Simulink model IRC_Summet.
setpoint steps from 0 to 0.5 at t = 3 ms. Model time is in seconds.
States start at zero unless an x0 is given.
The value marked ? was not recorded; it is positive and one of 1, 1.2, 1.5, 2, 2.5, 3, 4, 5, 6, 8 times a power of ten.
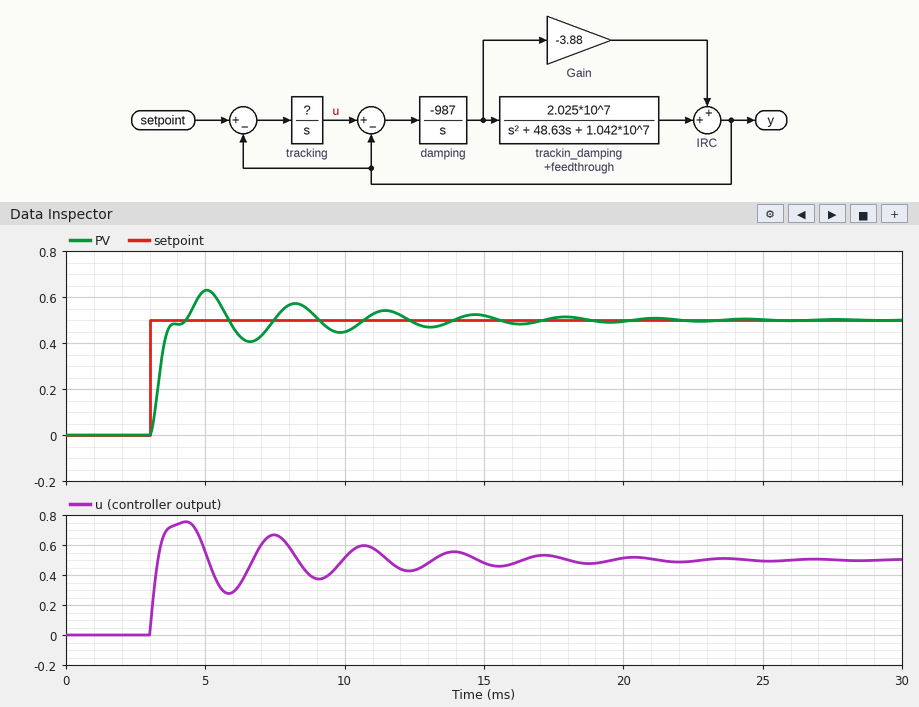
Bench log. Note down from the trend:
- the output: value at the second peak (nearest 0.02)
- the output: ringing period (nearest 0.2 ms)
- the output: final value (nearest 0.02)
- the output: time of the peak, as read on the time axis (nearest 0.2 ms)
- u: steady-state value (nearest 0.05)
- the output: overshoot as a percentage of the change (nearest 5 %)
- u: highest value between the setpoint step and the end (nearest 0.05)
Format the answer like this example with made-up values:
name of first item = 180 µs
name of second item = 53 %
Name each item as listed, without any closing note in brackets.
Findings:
the output: value at the second peak = 0.58
the output: ringing period = 3.2 ms
the output: final value = 0.50
the output: time of the peak, as read on the time axis = 5.0 ms
u: steady-state value = 0.50
the output: overshoot as a percentage of the change = 25 %
u: highest value between the setpoint step and the end = 0.75
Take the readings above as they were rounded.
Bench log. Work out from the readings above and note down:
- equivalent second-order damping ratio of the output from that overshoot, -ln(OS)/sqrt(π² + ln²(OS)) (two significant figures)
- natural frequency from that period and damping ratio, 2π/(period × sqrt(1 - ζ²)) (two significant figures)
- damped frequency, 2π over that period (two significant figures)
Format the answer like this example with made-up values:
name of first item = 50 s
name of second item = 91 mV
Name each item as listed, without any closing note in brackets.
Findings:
equivalent second-order damping ratio of the output from that overshoot, -ln(OS)/sqrt(π² + ln²(OS)) = 0.40
natural frequency from that period and damping ratio, 2π/(period × sqrt(1 - ζ²)) = 2.1 rad/ms
damped frequency, 2π over that period = 2.0 rad/ms
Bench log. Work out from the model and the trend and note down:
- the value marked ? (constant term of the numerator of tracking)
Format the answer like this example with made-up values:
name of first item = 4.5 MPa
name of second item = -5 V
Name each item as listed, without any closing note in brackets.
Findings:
the value marked ? = 4000
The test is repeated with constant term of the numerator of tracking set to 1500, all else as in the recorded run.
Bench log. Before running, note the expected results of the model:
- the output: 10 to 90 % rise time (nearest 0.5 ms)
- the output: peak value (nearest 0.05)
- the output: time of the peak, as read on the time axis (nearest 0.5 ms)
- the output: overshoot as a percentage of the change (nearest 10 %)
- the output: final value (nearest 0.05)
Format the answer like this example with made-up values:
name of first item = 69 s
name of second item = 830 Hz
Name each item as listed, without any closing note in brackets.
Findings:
the output: 10 to 90 % rise time = 1.5 ms
the output: peak value = 0.60
the output: time of the peak, as read on the time axis = 5.5 ms
the output: overshoot as a percentage of the change = 20 %
the output: final value = 0.50
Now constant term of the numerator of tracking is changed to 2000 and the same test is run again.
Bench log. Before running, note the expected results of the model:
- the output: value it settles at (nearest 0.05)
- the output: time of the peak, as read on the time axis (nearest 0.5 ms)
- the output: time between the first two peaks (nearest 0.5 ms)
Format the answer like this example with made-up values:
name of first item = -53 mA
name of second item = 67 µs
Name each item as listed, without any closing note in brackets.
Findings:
the output: value it settles at = 0.50
the output: time of the peak, as read on the time axis = 5.5 ms
the output: time between the first two peaks = 3.5 ms
